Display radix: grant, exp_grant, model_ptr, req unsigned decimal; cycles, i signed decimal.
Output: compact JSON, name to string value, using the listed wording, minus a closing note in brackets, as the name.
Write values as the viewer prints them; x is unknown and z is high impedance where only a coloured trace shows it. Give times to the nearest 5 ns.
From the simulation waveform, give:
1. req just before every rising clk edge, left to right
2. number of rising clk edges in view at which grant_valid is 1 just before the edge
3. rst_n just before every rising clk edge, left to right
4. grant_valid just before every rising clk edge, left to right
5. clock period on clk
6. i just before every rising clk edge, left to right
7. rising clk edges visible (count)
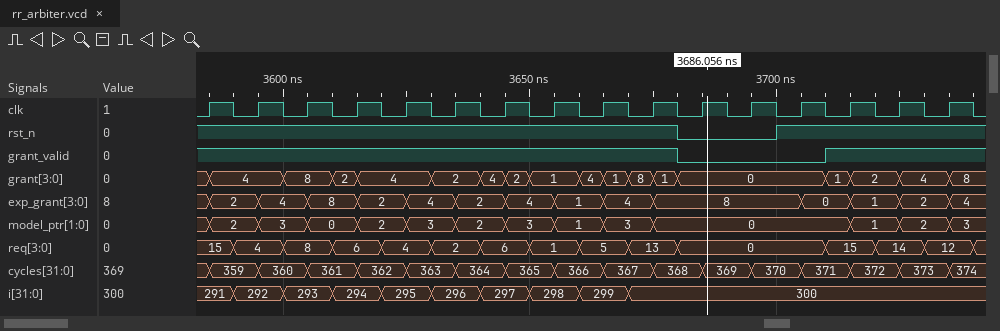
{"req just before every rising clk edge, left to right": "15, 4, 8, 6, 4, 2, 6, 1, 5, 13, 0, 0, 0, 15, 14, 12", "number of rising clk edges in view at which grant_valid is 1 just before the edge": "13", "rst_n just before every rising clk edge, left to right": "1 1 1 1 1 1 1 1 1 1 0 0 1 1 1 1", "grant_valid just before every rising clk edge, left to right": "1 1 1 1 1 1 1 1 1 1 0 0 0 1 1 1", "clock period on clk": "10 ns", "i just before every rising clk edge, left to right": "291, 292, 293, 294, 295, 296, 297, 298, 299, 300, 300, 300, 300, 300, 300, 300", "rising clk edges visible": "16"}
